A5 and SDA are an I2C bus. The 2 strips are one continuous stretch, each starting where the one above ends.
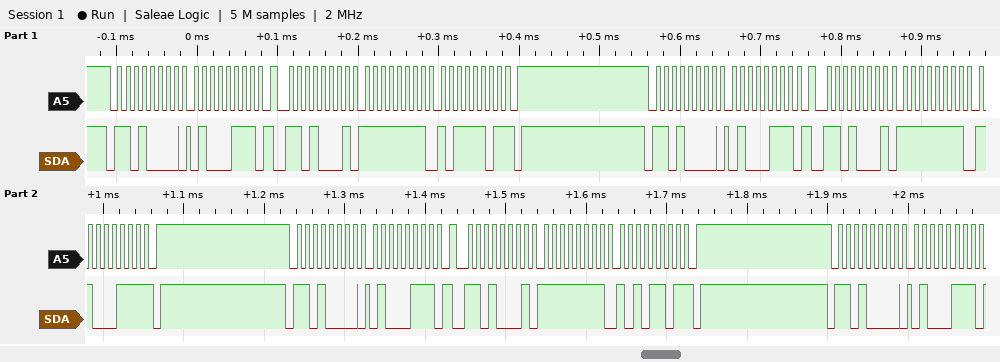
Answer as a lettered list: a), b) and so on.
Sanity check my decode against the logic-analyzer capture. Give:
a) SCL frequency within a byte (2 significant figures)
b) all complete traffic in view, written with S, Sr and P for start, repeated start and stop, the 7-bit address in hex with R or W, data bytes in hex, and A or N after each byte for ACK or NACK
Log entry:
a) 100 kHz
b) S 68W A 47 A Sr 68R A FF A BD N P S 68W A 47 A Sr 68R A FF A C7 N P S 68W A 47 A Sr 68R A FF A AD N P S 68W A 47 A
